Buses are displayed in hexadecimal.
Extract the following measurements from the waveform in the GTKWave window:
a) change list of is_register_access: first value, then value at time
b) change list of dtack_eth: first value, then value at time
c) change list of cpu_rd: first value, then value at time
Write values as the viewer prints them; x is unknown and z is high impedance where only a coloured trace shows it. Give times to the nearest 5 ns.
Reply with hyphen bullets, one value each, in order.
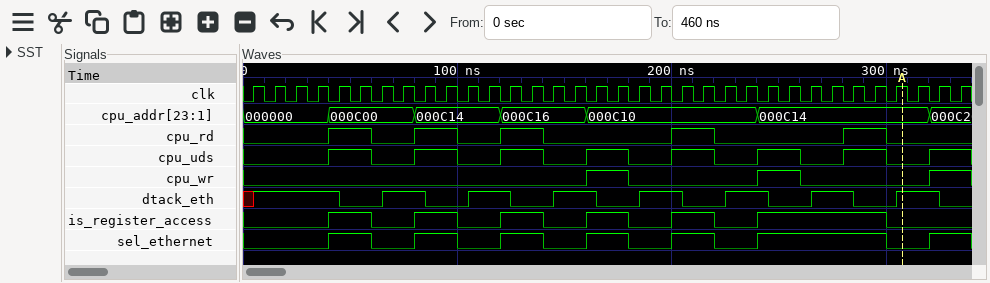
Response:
- 0, 1 at 40 ns, 0 at 60 ns, 1 at 80 ns, 0 at 100 ns, 1 at 120 ns, 0 at 140 ns, 1 at 160 ns, 0 at 180 ns, 1 at 200 ns, 0 at 220 ns, 1 at 240 ns, 0 at 300 ns
- x, 1 at 5 ns, 0 at 45 ns, 1 at 65 ns, 0 at 85 ns, 1 at 105 ns, 0 at 125 ns, 1 at 145 ns, 0 at 165 ns, 1 at 185 ns, 0 at 205 ns, 1 at 225 ns, 0 at 245 ns, 1 at 265 ns, 0 at 285 ns, 1 at 305 ns, 0 at 325 ns
- 0, 1 at 40 ns, 0 at 60 ns, 1 at 80 ns, 0 at 100 ns, 1 at 120 ns, 0 at 140 ns, 1 at 200 ns, 0 at 220 ns, 1 at 280 ns, 0 at 300 ns
